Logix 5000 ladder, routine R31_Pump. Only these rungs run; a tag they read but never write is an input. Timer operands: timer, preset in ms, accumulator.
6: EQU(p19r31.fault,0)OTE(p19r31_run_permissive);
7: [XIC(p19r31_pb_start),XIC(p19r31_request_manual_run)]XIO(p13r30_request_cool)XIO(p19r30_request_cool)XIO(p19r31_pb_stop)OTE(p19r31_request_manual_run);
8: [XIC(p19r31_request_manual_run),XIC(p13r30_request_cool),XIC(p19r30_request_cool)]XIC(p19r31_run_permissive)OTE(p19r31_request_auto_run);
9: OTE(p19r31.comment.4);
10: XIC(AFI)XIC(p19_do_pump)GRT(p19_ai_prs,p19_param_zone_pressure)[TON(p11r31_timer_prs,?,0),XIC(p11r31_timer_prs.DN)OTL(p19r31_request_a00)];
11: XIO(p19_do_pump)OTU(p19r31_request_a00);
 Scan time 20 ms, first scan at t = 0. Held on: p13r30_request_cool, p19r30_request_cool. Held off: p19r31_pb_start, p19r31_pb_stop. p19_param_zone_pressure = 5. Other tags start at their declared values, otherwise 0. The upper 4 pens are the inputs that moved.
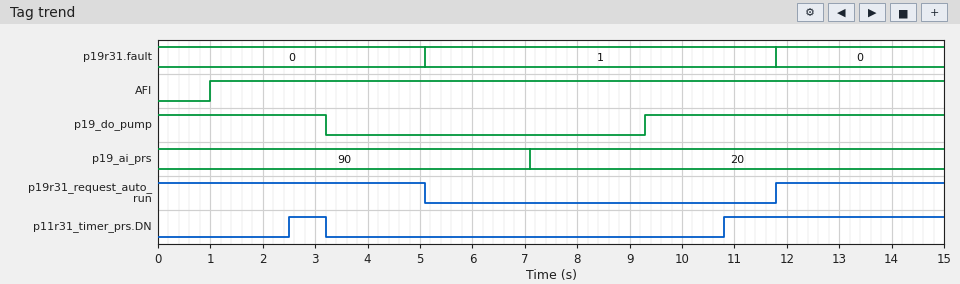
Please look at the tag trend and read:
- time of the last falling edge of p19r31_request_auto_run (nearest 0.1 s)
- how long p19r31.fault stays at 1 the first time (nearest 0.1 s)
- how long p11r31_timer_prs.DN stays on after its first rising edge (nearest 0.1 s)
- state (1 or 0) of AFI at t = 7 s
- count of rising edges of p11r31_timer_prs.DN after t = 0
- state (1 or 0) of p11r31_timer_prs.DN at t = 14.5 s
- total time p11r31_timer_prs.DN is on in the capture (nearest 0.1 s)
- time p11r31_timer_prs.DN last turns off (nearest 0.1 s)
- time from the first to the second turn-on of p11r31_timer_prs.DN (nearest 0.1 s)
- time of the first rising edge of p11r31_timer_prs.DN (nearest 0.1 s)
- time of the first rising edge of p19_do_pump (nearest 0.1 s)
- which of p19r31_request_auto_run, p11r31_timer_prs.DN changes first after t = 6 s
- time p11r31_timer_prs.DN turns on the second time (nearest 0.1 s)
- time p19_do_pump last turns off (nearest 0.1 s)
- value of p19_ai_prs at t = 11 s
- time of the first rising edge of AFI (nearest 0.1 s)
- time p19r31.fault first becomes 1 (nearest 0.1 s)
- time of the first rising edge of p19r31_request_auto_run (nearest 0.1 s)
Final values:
5.1 s
6.7 s
0.7 s
1
2
1
4.9 s
3.2 s
8.3 s
2.5 s
9.3 s
p11r31_timer_prs.DN
10.8 s
3.2 s
20
1.0 s
5.1 s
11.8 s
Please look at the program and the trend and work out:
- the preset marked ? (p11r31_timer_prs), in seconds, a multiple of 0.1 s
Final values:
1.5 s
